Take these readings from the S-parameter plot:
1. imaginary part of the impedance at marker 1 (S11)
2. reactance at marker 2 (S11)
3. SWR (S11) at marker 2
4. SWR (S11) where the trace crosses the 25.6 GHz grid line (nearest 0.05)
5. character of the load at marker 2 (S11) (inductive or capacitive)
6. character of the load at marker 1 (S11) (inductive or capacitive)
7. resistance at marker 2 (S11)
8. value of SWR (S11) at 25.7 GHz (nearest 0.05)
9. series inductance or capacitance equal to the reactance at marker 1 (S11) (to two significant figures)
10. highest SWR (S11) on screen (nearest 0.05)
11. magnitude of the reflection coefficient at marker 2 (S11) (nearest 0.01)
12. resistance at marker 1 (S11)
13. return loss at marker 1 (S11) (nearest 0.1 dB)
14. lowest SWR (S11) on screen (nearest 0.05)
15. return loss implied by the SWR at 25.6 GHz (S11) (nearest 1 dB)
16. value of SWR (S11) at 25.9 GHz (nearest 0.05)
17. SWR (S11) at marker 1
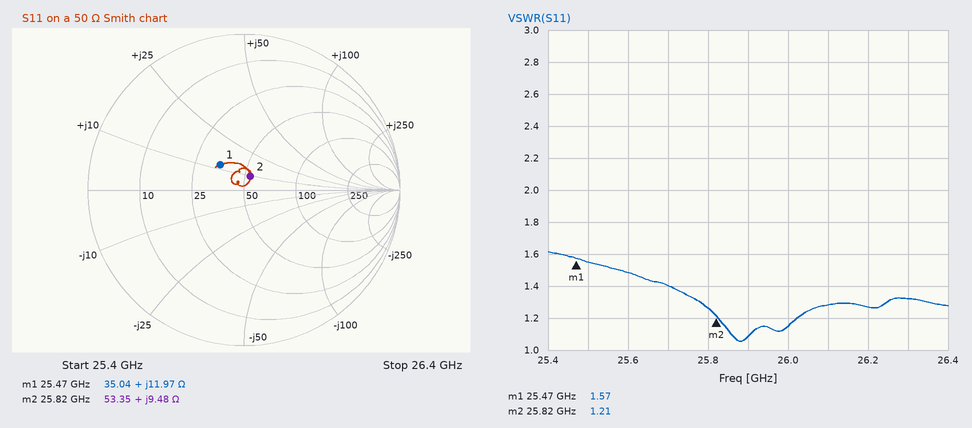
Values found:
+11.97 Ω
+9.48 Ω
1.21
1.50
inductive
inductive
53.35 Ω
1.40
75 pH
1.60
0.10
35.04 Ω
13.0 dB
1.05
14 dB
1.10
1.57
